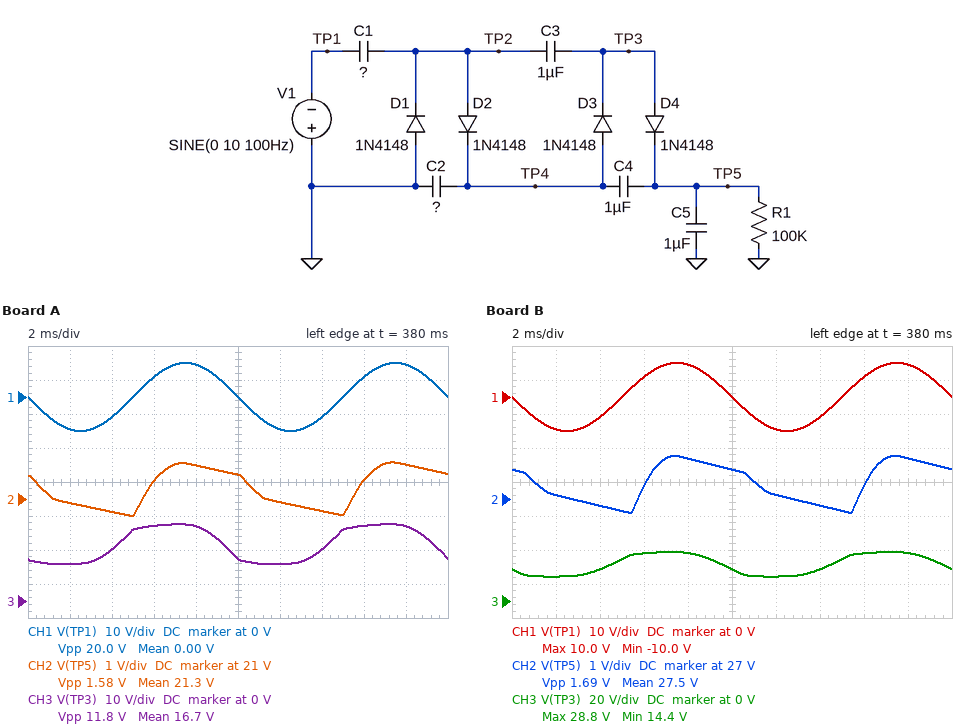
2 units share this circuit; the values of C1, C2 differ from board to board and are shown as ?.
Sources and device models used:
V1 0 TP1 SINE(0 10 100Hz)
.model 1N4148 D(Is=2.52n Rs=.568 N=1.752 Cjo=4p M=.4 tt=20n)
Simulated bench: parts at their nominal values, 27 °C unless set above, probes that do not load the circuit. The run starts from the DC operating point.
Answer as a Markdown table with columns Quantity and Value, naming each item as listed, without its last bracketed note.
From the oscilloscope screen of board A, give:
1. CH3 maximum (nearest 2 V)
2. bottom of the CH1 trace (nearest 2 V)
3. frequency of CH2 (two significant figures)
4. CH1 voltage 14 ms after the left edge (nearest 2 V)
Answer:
| Quantity | Value |
|---|---|
| CH3 maximum | 22 V |
| bottom of the CH1 trace | -10 V |
| frequency of CH2 | 100 Hz |
| CH1 voltage 14 ms after the left edge | -6 V |
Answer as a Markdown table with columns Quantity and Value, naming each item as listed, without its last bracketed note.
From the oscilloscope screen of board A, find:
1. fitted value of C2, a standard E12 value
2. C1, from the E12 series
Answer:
| Quantity | Value |
|---|---|
| fitted value of C2, a standard E12 value | 1.5 µF |
| C1, from the E12 series | 680 nF |
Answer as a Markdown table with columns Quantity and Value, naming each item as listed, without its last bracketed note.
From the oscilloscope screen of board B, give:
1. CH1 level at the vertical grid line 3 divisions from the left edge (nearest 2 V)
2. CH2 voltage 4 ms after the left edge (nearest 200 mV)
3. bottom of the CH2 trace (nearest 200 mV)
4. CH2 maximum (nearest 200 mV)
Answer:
| Quantity | Value |
|---|---|
| CH1 level at the vertical grid line 3 divisions from the left edge | 6 V |
| CH2 voltage 4 ms after the left edge | 26.8 V |
| bottom of the CH2 trace | 26.6 V |
| CH2 maximum | 28.2 V |
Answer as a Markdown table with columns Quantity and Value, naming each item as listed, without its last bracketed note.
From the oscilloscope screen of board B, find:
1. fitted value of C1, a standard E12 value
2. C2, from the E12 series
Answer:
| Quantity | Value |
|---|---|
| fitted value of C1, a standard E12 value | 1.8 µF |
| C2, from the E12 series | 2.7 µF |
